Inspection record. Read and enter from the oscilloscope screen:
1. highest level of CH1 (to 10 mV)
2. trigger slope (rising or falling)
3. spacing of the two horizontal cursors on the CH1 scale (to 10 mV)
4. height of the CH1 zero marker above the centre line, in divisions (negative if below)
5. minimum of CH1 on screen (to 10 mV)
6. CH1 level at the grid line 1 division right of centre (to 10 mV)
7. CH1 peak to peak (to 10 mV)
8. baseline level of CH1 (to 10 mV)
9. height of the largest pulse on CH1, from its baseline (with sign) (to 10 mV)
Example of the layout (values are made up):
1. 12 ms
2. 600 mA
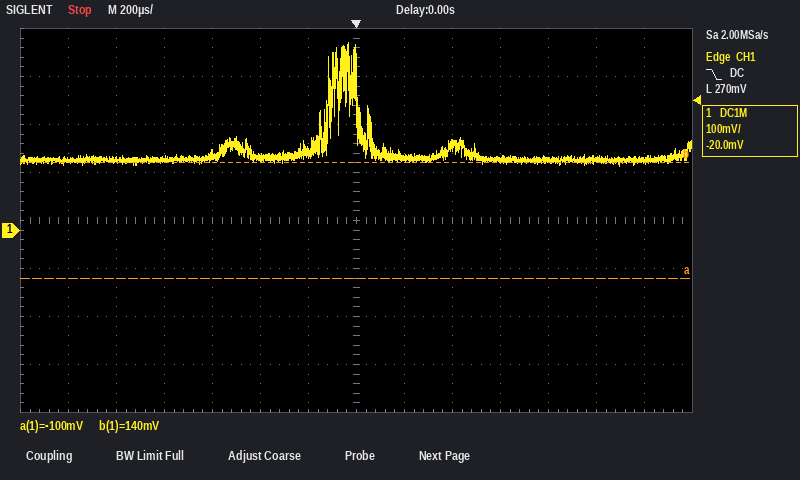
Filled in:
1. 390 mV
2. falling
3. 240 mV
4. -0.2 div
5. 130 mV
6. 150 mV
7. 260 mV
8. 150 mV
9. +240 mV
